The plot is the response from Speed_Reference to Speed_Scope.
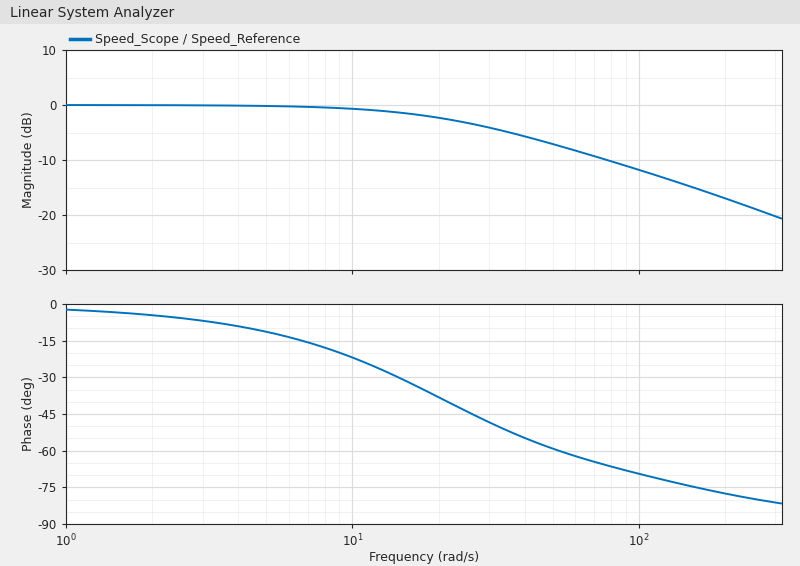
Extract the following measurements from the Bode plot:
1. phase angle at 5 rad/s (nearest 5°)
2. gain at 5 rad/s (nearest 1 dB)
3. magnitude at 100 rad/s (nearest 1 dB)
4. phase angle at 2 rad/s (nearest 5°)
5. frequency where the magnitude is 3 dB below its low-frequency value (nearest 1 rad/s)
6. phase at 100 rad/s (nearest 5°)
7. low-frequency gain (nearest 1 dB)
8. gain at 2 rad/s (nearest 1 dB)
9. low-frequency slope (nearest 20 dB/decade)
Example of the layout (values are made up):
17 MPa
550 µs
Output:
-10°
0 dB
-12 dB
-5°
24 rad/s
-70°
0 dB
0 dB
0 dB/decade
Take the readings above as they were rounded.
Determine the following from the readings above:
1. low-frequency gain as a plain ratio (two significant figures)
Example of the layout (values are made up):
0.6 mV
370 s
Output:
1.0
